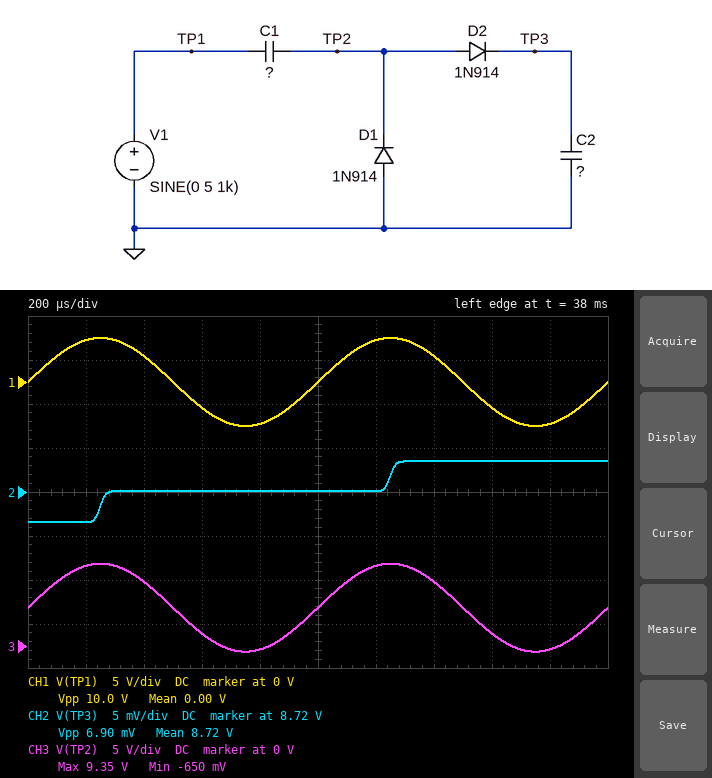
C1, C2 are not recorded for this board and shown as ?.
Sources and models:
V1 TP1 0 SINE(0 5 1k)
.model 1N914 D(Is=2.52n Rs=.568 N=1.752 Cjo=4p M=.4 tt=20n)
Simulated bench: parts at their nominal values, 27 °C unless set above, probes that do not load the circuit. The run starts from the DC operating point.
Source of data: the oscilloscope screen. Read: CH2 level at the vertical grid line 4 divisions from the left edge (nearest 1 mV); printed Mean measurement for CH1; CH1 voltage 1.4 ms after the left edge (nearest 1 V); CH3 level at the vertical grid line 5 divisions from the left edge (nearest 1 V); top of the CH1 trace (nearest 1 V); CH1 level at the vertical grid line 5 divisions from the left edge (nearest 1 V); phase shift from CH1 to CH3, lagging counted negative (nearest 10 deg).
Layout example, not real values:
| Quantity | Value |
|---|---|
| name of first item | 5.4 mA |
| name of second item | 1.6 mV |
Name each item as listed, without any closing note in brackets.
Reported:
| Quantity | Value |
|---|---|
| CH2 level at the vertical grid line 4 divisions from the left edge | 8.720 V |
| printed Mean measurement for CH1 | 0.00 V |
| CH1 voltage 1.4 ms after the left edge | 3 V |
| CH3 level at the vertical grid line 5 divisions from the left edge | 4 V |
| top of the CH1 trace | 5 V |
| CH1 level at the vertical grid line 5 divisions from the left edge | 0 V |
| phase shift from CH1 to CH3, lagging counted negative | 0 deg |
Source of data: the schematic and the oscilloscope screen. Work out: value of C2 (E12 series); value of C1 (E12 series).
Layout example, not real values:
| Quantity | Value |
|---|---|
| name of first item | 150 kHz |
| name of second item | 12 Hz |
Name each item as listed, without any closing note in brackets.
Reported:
| Quantity | Value |
|---|---|
| value of C2 | 33 µF |
| value of C1 | 15 µF |
